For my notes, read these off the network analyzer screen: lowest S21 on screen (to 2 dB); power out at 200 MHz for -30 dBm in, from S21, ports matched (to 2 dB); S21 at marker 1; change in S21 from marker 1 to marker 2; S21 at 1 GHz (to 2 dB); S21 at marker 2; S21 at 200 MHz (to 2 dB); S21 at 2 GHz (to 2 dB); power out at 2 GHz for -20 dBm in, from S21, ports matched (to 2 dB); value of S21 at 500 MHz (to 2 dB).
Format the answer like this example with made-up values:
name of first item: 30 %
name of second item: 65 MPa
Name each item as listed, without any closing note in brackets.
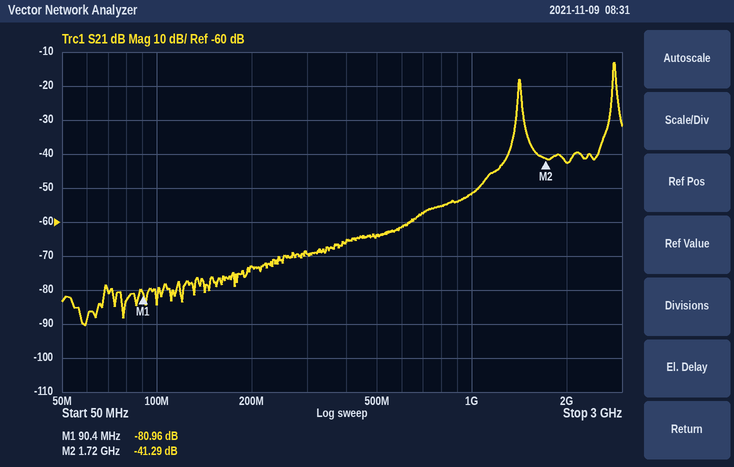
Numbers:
lowest S21 on screen: -90 dB
power out at 200 MHz for -30 dBm in, from S21, ports matched: -104 dBm
S21 at marker 1: -80.96 dB
change in S21 from marker 1 to marker 2: 39.67 dB
S21 at 1 GHz: -52 dB
S21 at marker 2: -41.29 dB
S21 at 200 MHz: -74 dB
S21 at 2 GHz: -42 dB
power out at 2 GHz for -20 dBm in, from S21, ports matched: -62 dBm
value of S21 at 500 MHz: -64 dB
